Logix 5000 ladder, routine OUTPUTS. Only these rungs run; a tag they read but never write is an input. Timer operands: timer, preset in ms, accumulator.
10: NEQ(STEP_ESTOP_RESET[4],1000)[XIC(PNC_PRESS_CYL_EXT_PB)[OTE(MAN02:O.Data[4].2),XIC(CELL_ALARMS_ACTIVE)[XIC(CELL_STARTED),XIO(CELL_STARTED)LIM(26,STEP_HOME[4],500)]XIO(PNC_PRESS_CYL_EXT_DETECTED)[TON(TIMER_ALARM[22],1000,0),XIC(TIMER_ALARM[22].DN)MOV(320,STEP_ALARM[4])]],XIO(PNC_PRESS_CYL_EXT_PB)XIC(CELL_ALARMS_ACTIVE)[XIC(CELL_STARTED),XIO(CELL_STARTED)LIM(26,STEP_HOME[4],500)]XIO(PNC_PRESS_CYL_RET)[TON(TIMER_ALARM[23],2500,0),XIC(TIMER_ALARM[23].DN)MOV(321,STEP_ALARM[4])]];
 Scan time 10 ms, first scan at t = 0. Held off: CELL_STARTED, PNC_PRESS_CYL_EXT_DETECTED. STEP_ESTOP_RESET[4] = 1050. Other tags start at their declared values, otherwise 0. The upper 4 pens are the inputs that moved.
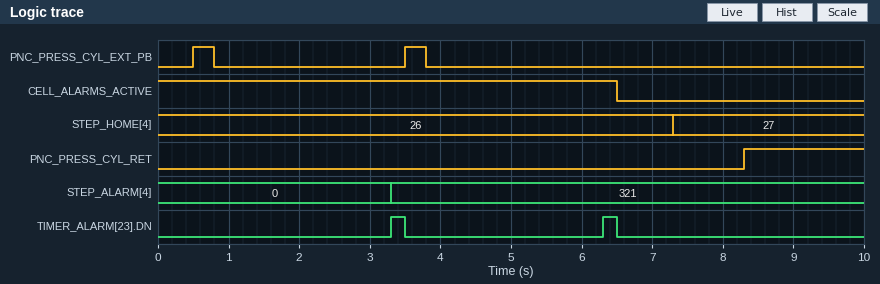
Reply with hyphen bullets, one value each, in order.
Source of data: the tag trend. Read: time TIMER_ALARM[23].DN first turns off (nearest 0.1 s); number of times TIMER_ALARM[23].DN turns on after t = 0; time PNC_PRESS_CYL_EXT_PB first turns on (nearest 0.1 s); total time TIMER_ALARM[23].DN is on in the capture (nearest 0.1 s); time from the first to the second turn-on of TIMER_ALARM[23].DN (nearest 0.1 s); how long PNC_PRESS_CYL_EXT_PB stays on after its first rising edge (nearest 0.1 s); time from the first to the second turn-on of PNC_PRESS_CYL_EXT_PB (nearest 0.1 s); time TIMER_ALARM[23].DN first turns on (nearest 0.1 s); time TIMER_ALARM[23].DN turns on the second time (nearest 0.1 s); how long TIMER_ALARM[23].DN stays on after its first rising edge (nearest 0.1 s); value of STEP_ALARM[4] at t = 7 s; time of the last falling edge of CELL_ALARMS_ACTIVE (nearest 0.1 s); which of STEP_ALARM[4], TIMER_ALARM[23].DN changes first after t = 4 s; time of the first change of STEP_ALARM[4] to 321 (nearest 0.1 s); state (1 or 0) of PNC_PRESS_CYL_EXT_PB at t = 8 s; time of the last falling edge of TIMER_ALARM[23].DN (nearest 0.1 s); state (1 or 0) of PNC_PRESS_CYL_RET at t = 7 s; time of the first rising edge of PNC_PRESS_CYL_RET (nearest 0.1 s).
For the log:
- 3.5 s
- 2
- 0.5 s
- 0.4 s
- 3.0 s
- 0.3 s
- 3.0 s
- 3.3 s
- 6.3 s
- 0.2 s
- 321
- 6.5 s
- TIMER_ALARM[23].DN
- 3.3 s
- 0
- 6.5 s
- 0
- 8.3 s
